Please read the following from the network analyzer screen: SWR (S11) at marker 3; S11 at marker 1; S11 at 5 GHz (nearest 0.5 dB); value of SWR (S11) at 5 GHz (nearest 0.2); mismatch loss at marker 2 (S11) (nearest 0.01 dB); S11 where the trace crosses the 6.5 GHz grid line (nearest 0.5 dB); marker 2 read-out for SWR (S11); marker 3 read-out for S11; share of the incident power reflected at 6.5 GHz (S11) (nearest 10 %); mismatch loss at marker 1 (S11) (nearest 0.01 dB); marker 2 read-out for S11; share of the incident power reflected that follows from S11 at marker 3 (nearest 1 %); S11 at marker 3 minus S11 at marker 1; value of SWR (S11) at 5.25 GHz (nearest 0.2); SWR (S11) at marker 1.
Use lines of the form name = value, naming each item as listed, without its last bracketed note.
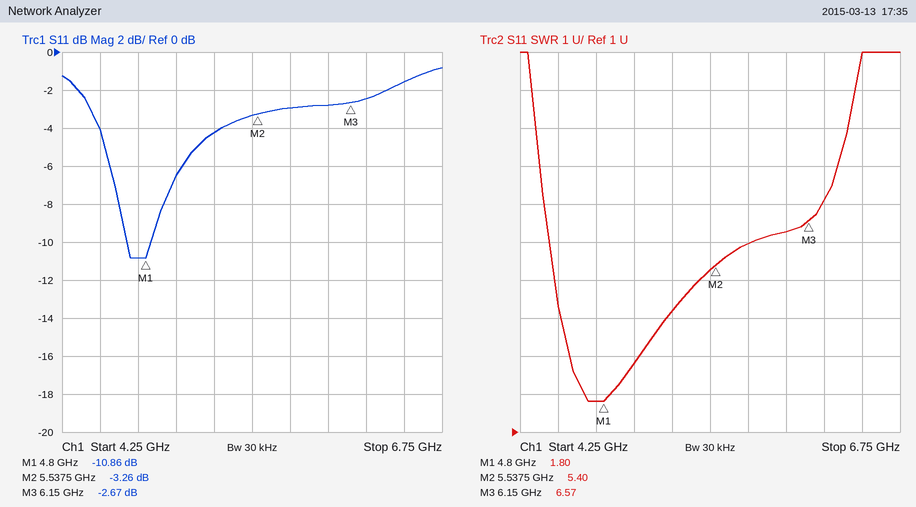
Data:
SWR (S11) at marker 3 = 6.57
S11 at marker 1 = -10.86 dB
S11 at 5 GHz = -6.5 dB
value of SWR (S11) at 5 GHz = 2.8
mismatch loss at marker 2 (S11) = 2.77 dB
S11 where the trace crosses the 6.5 GHz grid line = -1.5 dB
marker 2 read-out for SWR = 5.40
marker 3 read-out for S11 = -2.67 dB
share of the incident power reflected at 6.5 GHz (S11) = 70 %
mismatch loss at marker 1 (S11) = 0.37 dB
marker 2 read-out for S11 = -3.26 dB
share of the incident power reflected that follows from S11 at marker 3 = 54 %
S11 at marker 3 minus S11 at marker 1 = 8.19 dB
value of SWR (S11) at 5.25 GHz = 4.2
SWR (S11) at marker 1 = 1.80
